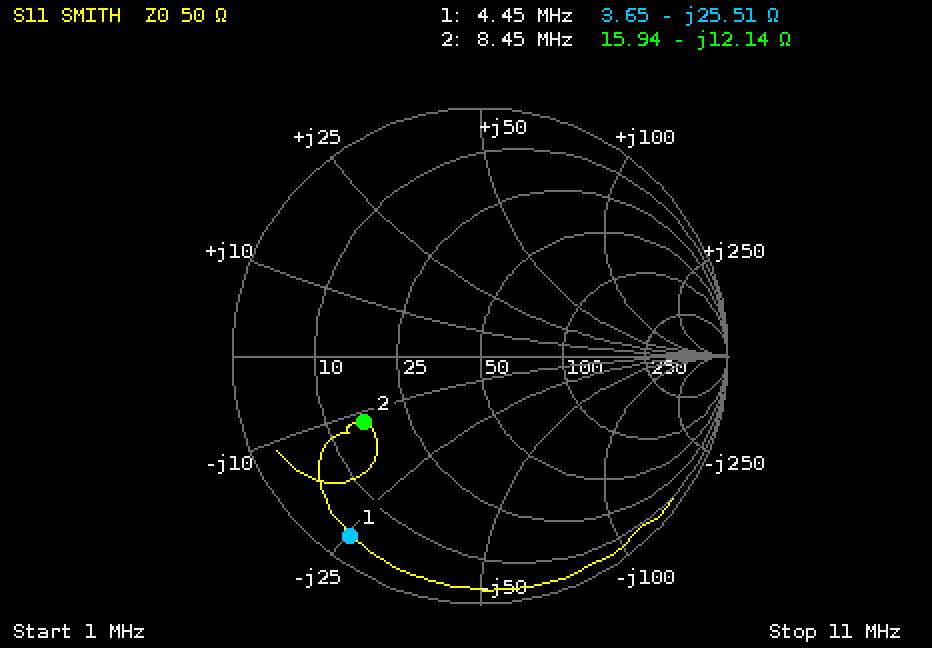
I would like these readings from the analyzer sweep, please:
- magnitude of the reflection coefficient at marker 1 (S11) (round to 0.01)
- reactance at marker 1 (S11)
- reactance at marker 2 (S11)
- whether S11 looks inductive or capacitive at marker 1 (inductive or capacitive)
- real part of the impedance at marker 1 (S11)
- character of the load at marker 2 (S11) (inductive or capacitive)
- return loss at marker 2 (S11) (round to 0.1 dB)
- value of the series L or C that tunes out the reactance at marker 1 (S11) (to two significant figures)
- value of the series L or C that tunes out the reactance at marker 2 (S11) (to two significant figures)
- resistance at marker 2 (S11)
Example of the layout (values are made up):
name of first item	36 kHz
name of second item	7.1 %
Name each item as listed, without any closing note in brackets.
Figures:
magnitude of the reflection coefficient at marker 1 (S11)	0.89
reactance at marker 1	-25.51 Ω
reactance at marker 2	-12.14 Ω
whether S11 looks inductive or capacitive at marker 1	capacitive
real part of the impedance at marker 1	3.65 Ω
character of the load at marker 2 (S11)	capacitive
return loss at marker 2 (S11)	5.4 dB
value of the series L or C that tunes out the reactance at marker 1 (S11)	910 nH
value of the series L or C that tunes out the reactance at marker 2 (S11)	230 nH
resistance at marker 2	15.94 Ω
